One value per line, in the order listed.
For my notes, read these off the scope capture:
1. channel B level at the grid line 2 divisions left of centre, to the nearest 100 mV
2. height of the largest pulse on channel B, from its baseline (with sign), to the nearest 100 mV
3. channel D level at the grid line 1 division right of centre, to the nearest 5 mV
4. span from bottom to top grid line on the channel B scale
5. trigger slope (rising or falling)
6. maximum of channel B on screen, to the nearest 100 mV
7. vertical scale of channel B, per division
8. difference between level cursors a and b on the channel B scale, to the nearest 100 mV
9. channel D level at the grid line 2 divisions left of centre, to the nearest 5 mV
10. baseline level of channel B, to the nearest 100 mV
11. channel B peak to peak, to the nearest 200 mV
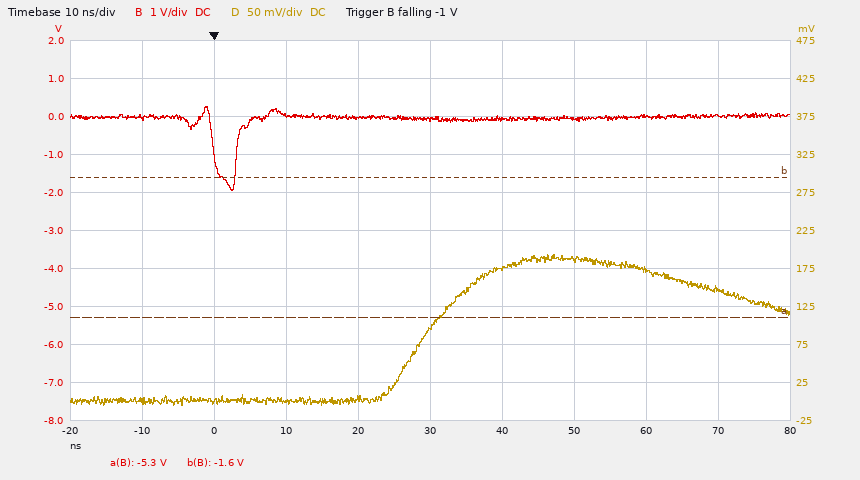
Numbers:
0.0 V
-1.9 V
175 mV
10 V
falling
300 mV
1 V
3.7 V
0 mV
0.0 V
2.2 V
